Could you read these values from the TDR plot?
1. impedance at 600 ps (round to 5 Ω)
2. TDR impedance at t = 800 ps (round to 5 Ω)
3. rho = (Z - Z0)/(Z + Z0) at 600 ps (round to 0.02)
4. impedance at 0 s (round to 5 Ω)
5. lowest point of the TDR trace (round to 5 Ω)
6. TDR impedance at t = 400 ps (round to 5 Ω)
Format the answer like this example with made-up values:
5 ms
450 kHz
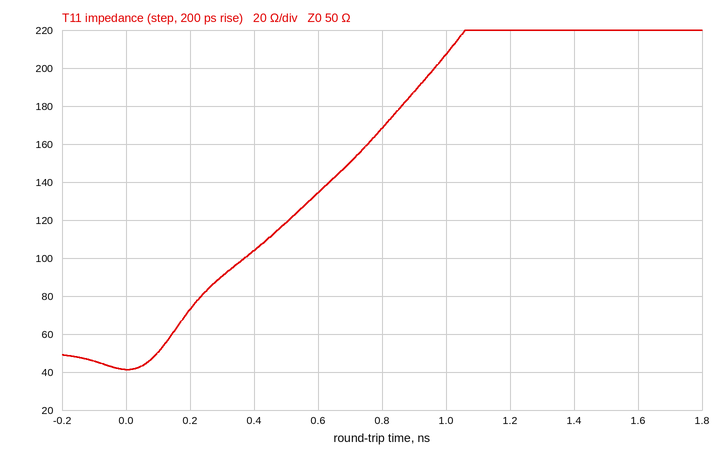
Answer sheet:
135 Ω
170 Ω
+0.46
40 Ω
40 Ω
105 Ω
